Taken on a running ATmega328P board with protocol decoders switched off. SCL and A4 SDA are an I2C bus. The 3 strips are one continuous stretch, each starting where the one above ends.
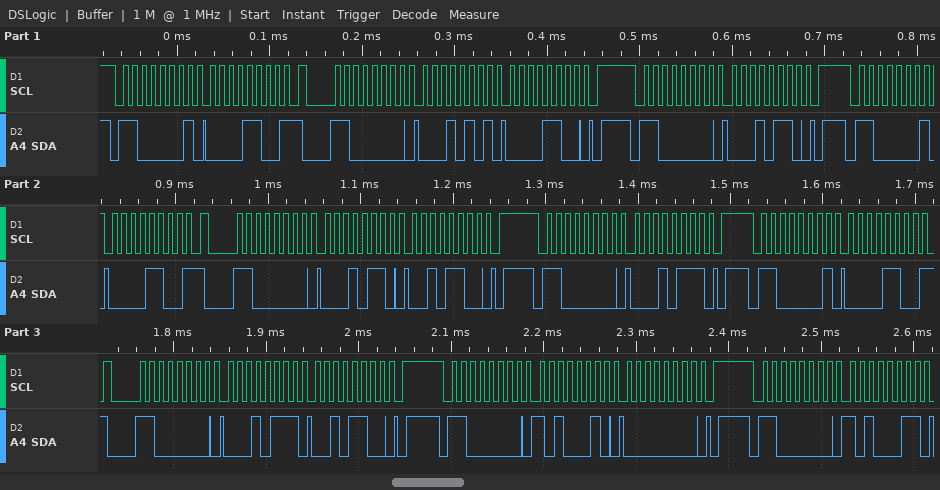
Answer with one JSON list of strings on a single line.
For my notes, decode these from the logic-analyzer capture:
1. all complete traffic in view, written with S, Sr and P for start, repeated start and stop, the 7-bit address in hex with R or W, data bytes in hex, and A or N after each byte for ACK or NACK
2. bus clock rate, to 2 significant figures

["S 60R A 0C N Sr 60W A 15 A 0C A P S 60W A 16 A P S 60R A 0C N Sr 60W A 16 A 2C A P S 60W A 17 A P S 60R A 0C N Sr 60W A 17 A 2C A P S 60W A A2 A 00 A P S 60W A A3 A", "100 kHz"]
